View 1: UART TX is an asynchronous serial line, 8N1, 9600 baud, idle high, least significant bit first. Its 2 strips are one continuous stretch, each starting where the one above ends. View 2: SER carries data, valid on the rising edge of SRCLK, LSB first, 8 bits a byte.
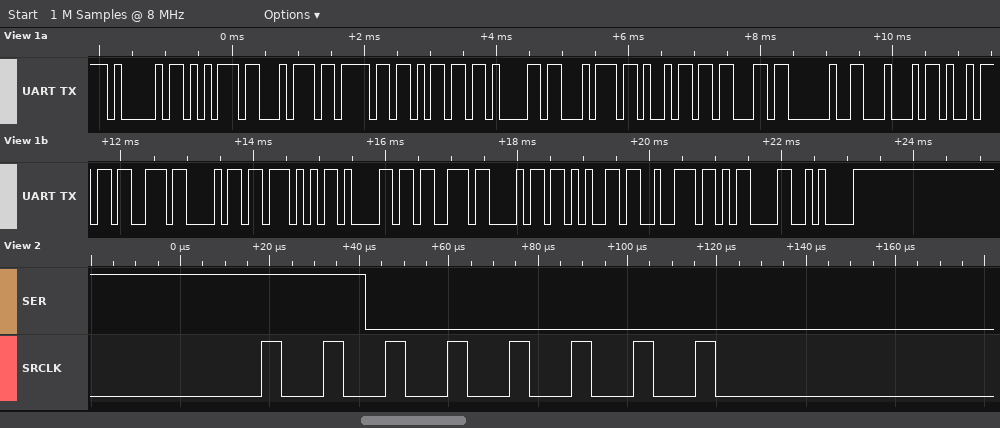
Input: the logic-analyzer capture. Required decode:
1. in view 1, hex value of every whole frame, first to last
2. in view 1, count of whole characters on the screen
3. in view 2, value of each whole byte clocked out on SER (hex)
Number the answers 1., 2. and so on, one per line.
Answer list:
1. 41 75 74 6F 6D 61 74 69 63 20 44 69 73 68 57 61 73 68 65 72 0D 0A
2. 22
3. 03
